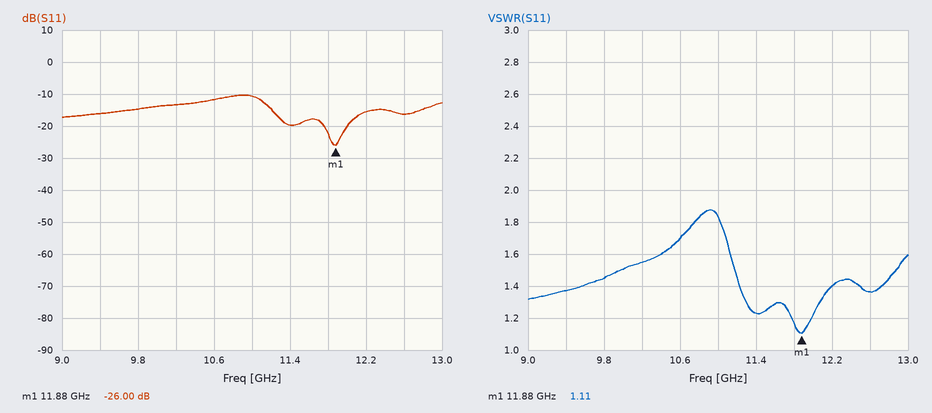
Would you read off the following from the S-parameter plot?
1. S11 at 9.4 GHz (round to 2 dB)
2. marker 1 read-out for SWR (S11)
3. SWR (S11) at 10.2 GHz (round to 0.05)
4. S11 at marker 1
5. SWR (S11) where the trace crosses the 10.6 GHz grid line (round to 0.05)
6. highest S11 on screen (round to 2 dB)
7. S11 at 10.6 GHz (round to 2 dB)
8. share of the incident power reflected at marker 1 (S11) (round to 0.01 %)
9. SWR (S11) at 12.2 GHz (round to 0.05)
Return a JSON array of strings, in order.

["-16 dB", "1.11", "1.55", "-26.00 dB", "1.70", "-10 dB", "-12 dB", "0.25 %", "1.40"]
